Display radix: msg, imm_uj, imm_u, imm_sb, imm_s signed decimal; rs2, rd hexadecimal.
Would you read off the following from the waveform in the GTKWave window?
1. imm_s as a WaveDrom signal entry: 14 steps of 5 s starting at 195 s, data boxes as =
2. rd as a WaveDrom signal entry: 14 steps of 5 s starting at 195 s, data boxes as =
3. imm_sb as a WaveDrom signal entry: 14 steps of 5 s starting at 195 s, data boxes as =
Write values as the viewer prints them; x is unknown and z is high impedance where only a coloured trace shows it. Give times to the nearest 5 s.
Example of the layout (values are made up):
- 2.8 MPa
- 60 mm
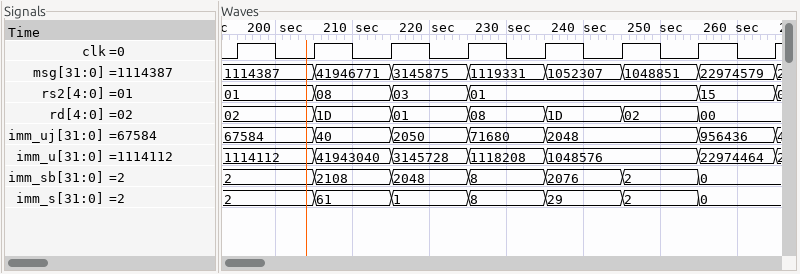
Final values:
- {name: 'imm_s', wave: '=.=.=.=.=.=.=.', data: '2 61 1 8 29 2 0'}
- {name: 'rd', wave: '=.=.=.=.=.=.=.', data: '02 1D 01 08 1D 02 00'}
- {name: 'imm_sb', wave: '=.=.=.=.=.=.=.', data: '2 2108 2048 8 2076 2 0'}
